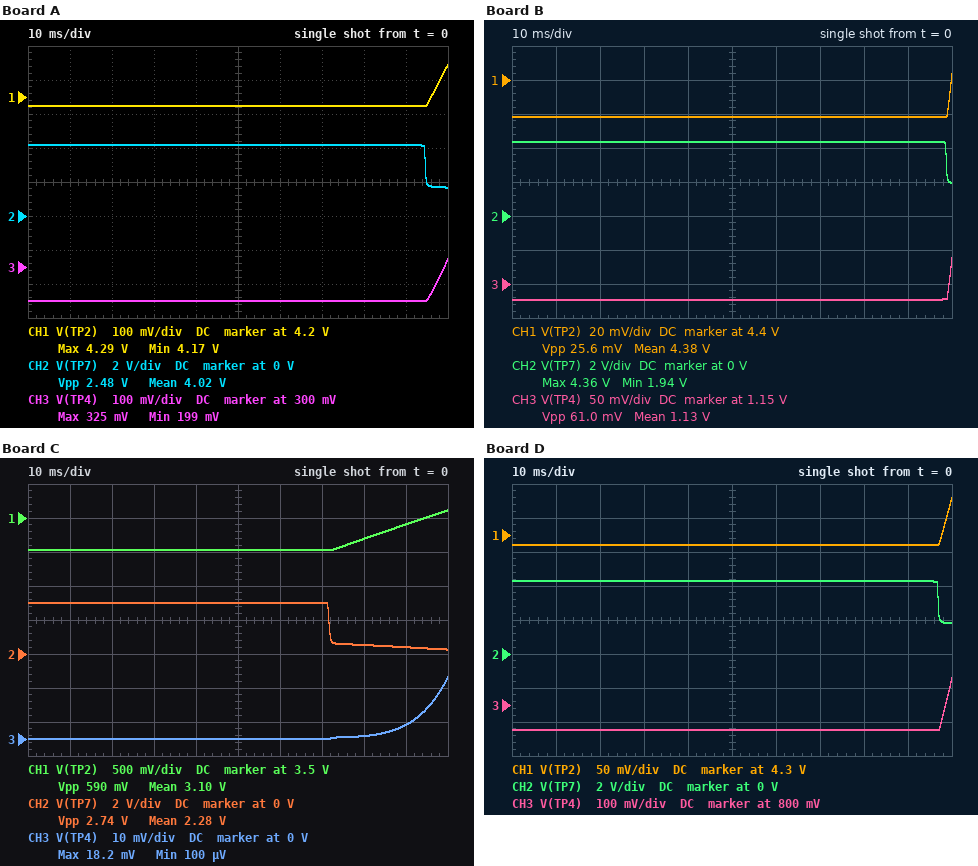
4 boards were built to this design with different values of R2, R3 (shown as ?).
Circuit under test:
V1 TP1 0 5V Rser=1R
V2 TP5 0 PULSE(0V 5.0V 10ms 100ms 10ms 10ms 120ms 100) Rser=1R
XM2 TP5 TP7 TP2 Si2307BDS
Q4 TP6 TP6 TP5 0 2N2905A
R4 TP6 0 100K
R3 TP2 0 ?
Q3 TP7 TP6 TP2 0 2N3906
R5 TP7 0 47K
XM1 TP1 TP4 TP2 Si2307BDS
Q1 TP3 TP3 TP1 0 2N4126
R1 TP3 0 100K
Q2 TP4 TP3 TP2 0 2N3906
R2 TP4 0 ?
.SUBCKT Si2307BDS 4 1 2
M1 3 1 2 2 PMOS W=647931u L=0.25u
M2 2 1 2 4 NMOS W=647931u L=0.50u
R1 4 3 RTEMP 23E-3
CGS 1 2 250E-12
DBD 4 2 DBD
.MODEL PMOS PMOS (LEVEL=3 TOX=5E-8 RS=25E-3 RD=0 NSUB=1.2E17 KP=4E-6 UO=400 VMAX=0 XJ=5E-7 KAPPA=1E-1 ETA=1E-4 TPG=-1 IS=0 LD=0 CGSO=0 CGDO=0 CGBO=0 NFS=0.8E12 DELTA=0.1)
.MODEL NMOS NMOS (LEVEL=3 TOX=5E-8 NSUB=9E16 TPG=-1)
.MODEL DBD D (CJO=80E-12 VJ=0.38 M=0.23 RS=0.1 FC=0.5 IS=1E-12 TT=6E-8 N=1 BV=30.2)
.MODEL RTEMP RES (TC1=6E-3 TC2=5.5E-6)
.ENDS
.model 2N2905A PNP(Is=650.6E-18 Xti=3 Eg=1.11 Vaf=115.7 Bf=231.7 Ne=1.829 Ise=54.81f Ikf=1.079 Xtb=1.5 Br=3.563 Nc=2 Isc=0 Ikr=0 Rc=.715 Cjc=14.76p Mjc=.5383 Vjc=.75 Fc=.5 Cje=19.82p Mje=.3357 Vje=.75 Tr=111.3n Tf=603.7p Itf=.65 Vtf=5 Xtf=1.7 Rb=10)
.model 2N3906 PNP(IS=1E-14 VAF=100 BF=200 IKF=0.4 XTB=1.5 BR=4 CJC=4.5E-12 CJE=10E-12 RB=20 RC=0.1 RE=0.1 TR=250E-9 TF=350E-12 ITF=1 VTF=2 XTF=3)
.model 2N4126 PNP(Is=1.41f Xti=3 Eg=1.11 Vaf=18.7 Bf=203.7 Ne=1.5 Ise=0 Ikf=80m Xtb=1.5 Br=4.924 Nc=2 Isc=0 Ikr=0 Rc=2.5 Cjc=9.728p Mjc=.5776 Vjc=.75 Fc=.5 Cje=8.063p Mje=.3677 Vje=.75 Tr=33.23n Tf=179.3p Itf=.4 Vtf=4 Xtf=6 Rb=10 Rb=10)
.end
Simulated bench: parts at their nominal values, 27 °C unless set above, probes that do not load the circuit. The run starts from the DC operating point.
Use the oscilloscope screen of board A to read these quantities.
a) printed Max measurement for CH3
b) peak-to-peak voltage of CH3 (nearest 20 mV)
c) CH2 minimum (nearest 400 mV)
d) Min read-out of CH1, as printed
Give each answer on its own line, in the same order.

325 mV
120 mV
1.6 V
4.17 V
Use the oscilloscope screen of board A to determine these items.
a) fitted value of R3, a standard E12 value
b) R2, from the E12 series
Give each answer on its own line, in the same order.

5.6 Ω
18 kΩ
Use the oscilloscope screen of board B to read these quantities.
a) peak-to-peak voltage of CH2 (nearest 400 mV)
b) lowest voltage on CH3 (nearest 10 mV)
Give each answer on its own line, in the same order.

2.4 V
1.13 V
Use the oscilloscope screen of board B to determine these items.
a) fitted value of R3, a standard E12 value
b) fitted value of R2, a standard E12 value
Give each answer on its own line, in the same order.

8.2 Ω
120 kΩ
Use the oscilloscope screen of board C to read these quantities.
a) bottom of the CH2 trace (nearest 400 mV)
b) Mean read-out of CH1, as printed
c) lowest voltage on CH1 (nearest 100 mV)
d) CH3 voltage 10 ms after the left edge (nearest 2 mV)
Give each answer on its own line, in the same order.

400 mV
3.10 V
3.0 V
0 V
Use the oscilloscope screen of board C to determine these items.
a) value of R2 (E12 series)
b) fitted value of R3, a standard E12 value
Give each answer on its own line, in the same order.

33 kΩ
1.8 Ω
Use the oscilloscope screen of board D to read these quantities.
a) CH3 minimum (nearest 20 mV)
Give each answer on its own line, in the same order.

720 mV
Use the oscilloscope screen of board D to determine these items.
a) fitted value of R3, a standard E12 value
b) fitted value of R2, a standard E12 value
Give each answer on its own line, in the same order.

6.8 Ω
68 kΩ
